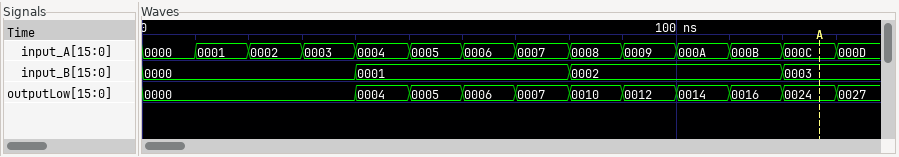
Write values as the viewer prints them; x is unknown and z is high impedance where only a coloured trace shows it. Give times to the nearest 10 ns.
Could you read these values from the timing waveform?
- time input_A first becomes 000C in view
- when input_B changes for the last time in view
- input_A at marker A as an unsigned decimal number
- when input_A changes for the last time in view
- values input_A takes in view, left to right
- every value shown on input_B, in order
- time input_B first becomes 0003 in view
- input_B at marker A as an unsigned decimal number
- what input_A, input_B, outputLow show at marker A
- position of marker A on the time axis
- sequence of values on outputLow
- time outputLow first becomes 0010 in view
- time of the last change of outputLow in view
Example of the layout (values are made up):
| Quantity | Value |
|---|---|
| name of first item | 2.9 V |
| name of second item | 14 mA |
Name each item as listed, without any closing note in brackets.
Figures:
| Quantity | Value |
|---|---|
| time input_A first becomes 000C in view | 120 ns |
| when input_B changes for the last time in view | 120 ns |
| input_A at marker A as an unsigned decimal number | 12 |
| when input_A changes for the last time in view | 130 ns |
| values input_A takes in view, left to right | 0000, 0001, 0002, 0003, 0004, 0005, 0006, 0007, 0008, 0009, 000A, 000B, 000C, 000D |
| every value shown on input_B, in order | 0000, 0001, 0002, 0003 |
| time input_B first becomes 0003 in view | 120 ns |
| input_B at marker A as an unsigned decimal number | 3 |
| what input_A, input_B, outputLow show at marker A | input_A=000C, input_B=0003, outputLow=0024 |
| position of marker A on the time axis | 130 ns |
| sequence of values on outputLow | 0000, 0004, 0005, 0006, 0007, 0010, 0012, 0014, 0016, 0024, 0027 |
| time outputLow first becomes 0010 in view | 80 ns |
| time of the last change of outputLow in view | 130 ns |
